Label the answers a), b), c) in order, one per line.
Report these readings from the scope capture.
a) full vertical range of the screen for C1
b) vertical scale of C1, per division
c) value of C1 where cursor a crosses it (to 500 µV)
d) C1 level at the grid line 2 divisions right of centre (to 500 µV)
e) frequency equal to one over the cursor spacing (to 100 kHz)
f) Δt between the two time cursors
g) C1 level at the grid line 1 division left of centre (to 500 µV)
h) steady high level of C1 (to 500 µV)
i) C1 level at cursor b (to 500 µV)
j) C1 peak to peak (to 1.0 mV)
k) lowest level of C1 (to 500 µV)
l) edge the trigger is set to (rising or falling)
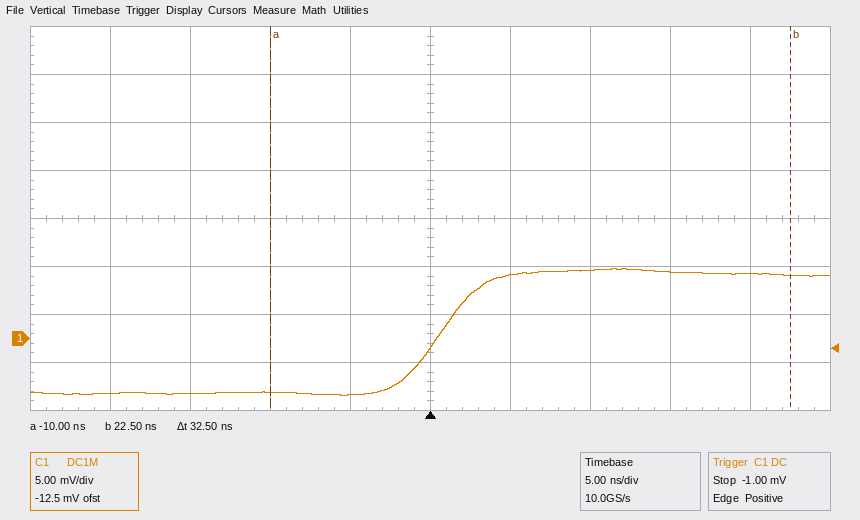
a) 40 mV
b) 5 mV
c) -5.5 mV
d) 7.0 mV
e) 30.8 MHz
f) 32.5 ns
g) -6.0 mV
h) 7.0 mV
i) 6.5 mV
j) 13.0 mV
k) -6.0 mV
l) rising
